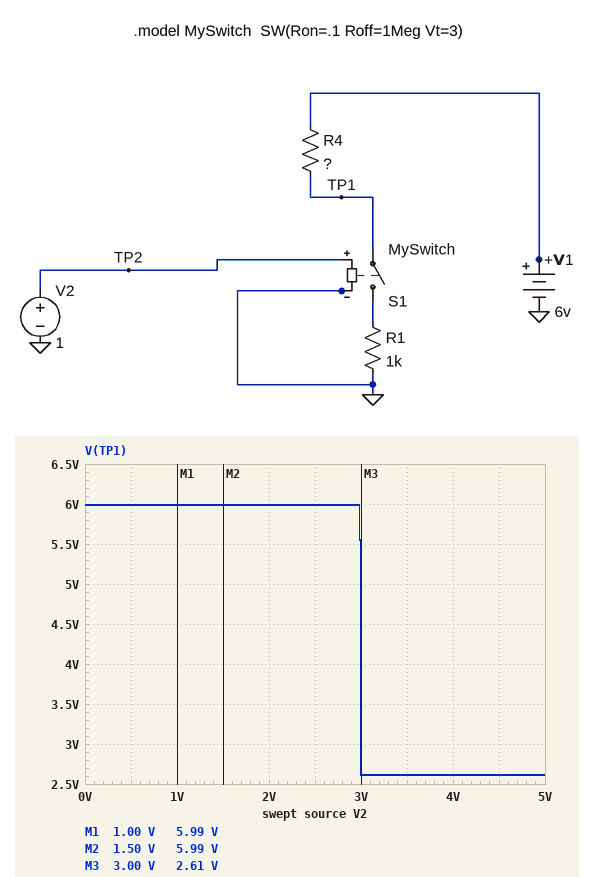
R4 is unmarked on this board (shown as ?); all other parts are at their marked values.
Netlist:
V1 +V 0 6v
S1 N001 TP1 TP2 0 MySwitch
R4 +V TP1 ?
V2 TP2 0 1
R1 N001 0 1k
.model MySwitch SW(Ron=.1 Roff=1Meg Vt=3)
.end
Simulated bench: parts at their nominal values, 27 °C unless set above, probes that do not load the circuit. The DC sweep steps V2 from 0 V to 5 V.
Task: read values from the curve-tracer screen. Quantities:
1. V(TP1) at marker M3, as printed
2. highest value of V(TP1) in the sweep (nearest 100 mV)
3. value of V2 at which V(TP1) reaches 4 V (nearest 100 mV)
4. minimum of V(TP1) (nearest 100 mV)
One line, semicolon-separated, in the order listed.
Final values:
2.61 V; 6.0 V; 3.0 V; 2.6 V
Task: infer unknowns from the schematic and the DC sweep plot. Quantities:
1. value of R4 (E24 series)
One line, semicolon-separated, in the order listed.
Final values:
1.3 kΩ
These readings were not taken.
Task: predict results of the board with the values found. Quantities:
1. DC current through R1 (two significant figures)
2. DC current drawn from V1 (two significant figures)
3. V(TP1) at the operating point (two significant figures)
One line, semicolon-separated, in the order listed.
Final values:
6.0 µA; 6.0 µA; 6.0 V
